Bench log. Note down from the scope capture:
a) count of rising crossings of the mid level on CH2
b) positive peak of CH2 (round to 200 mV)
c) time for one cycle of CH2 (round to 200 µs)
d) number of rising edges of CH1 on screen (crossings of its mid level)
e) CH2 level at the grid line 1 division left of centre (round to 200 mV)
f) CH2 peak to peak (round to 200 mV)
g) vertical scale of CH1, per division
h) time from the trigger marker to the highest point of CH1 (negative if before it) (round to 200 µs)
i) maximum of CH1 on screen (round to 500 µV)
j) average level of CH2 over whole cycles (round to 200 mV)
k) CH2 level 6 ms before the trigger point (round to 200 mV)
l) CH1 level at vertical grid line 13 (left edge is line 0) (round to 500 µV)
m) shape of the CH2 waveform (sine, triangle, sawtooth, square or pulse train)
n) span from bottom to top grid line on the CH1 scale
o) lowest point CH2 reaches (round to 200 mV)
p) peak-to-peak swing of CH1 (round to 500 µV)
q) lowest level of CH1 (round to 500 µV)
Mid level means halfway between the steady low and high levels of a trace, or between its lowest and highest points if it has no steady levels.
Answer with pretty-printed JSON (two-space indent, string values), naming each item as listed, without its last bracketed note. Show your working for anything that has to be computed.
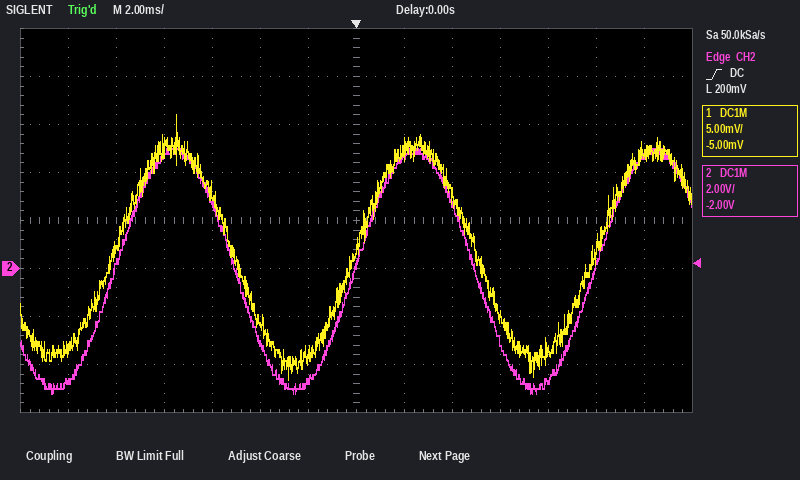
{
  "count of rising crossings of the mid level on CH2": "3",
  "positive peak of CH2": "5.0 V",
  "time for one cycle of CH2": "10.0 ms",
  "number of rising edges of CH1 on screen": "3",
  "CH2 level at the grid line 1 division left of centre": "-4.6 V",
  "CH2 peak to peak": "5.0 V − (-5.2 V) = 10.2 V",
  "vertical scale of CH1, per division": "5 mV",
  "time from the trigger marker to the highest point of CH1 (negative if before it)": "-7.4 ms",
  "maximum of CH1 on screen": "16.0 mV",
  "average level of CH2 over whole cycles": "(5.0 V + (-5.2 V)) / 2 ≈ 0.0 V",
  "CH2 level 6 ms before the trigger point": "2.6 V",
  "CH1 level at vertical grid line 13 (left edge is line 0)": "12.0 mV",
  "shape of the CH2 waveform": "sine",
  "span from bottom to top grid line on the CH1 scale": "40 mV",
  "lowest point CH2 reaches": "-5.2 V",
  "peak-to-peak swing of CH1": "16.0 mV − (-11.5 mV) = 27.5 mV",
  "lowest level of CH1": "-11.5 mV"
}
